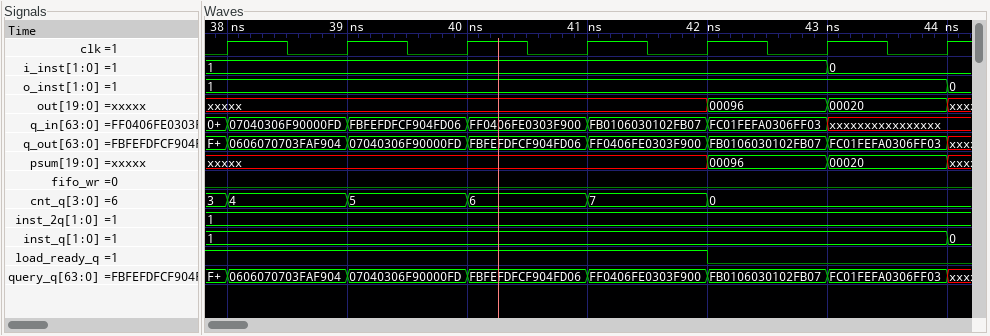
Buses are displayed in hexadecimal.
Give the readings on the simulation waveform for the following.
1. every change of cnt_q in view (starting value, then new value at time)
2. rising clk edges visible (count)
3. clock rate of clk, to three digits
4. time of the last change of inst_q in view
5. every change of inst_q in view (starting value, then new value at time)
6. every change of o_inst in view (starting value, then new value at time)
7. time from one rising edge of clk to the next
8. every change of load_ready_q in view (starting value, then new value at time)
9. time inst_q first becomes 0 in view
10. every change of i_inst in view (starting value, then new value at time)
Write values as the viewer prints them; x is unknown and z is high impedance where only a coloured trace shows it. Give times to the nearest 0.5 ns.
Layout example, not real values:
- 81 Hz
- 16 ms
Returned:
- 3, 4 at 38 ns, 5 at 39 ns, 6 at 40 ns, 7 at 41 ns, 0 at 42 ns
- 7
- 1.00 GHz
- 44 ns
- 1, 0 at 44 ns
- 1, 0 at 44 ns
- 1 ns
- 1, 0 at 42 ns
- 44 ns
- 1, 0 at 43 ns
